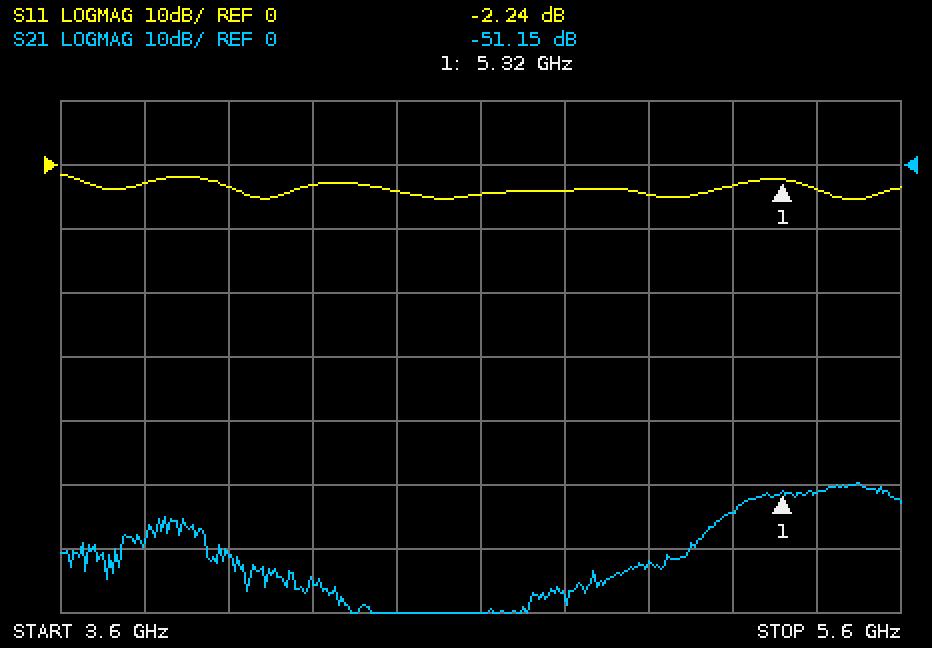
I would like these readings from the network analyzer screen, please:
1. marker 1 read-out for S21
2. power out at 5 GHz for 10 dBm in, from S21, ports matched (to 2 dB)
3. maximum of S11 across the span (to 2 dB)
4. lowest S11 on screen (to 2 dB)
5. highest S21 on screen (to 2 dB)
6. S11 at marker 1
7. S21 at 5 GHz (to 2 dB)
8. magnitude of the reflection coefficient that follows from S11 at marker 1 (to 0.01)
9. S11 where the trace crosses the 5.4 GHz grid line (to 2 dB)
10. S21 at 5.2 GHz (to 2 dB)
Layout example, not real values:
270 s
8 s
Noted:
-51.15 dB
-52 dBm
-2 dB
-6 dB
-50 dB
-2.24 dB
-62 dB
0.77
-4 dB
-54 dB
